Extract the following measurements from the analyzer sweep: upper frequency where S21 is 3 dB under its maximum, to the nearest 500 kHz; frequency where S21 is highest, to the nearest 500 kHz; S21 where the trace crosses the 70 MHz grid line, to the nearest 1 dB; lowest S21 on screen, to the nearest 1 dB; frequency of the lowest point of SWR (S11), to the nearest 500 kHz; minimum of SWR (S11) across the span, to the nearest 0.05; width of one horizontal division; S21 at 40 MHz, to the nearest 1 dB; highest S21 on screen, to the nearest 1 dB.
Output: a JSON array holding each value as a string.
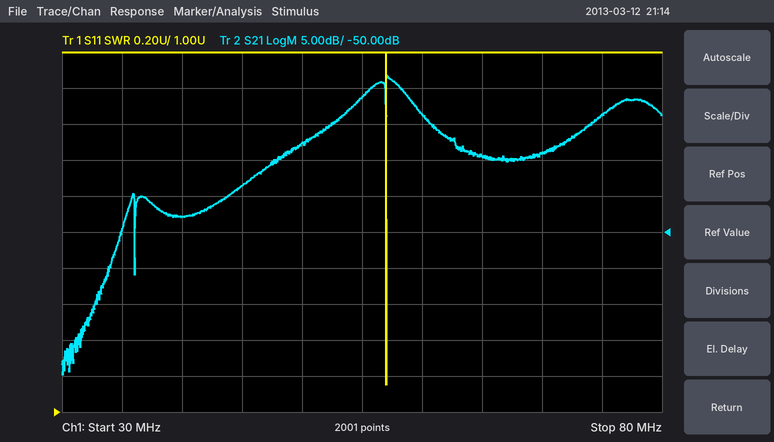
["59.0 MHz", "57.0 MHz", "-39 dB", "-70 dB", "57.0 MHz", "1.15", "5 MHz", "-48 dB", "-28 dB"]
